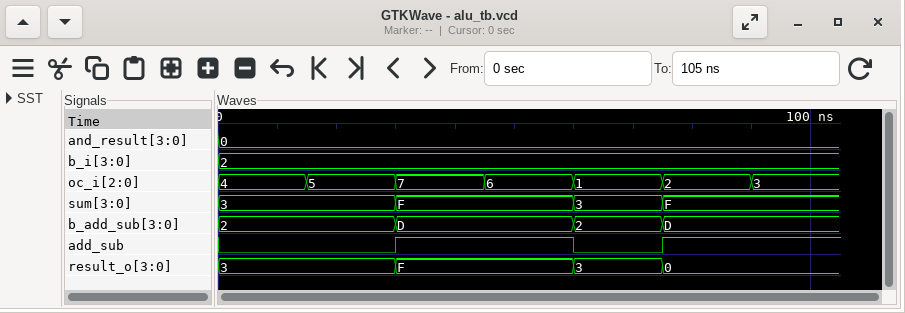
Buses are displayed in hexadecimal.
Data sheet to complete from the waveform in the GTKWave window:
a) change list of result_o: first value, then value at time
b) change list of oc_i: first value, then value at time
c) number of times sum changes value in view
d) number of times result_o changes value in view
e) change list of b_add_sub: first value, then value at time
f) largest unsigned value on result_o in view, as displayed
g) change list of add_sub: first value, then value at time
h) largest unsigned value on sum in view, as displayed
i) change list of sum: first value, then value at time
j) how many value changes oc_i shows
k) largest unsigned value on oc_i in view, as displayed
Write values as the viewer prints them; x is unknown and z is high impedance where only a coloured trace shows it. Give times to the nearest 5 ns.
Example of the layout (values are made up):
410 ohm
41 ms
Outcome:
3, F at 30 ns, 3 at 60 ns, 0 at 75 ns
4, 5 at 15 ns, 7 at 30 ns, 6 at 45 ns, 1 at 60 ns, 2 at 75 ns, 3 at 90 ns
3
3
2, D at 30 ns, 2 at 60 ns, D at 75 ns
F
0, 1 at 30 ns, 0 at 60 ns, 1 at 75 ns
F
3, F at 30 ns, 3 at 60 ns, F at 75 ns
6
7
